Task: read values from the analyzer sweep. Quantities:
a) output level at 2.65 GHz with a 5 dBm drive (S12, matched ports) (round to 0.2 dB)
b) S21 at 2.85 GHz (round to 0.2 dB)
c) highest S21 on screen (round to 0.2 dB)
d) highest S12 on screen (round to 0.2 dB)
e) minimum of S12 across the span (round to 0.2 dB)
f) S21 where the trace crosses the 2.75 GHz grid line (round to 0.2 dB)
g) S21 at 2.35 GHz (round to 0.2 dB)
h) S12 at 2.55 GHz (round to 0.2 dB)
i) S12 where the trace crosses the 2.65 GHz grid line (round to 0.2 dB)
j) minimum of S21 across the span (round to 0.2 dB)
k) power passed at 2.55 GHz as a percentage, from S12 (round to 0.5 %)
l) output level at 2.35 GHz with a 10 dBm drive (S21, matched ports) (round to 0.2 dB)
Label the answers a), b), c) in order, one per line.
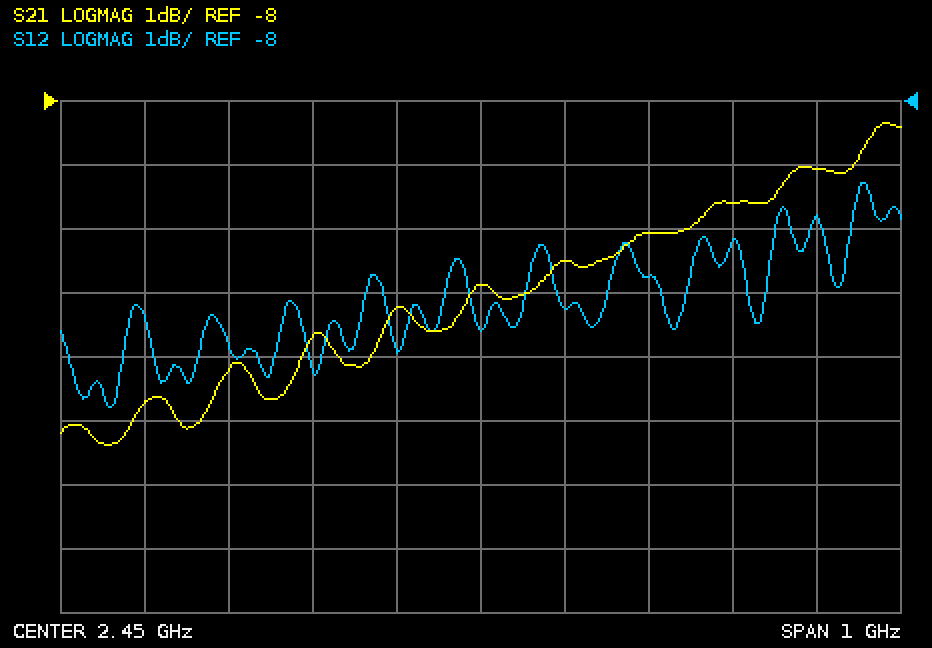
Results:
a) -5.8 dBm
b) -9.0 dB
c) -8.4 dB
d) -9.2 dB
e) -12.8 dB
f) -9.6 dB
g) -11.2 dB
h) -11.2 dB
i) -10.8 dB
j) -13.4 dB
k) 7.5 %
l) -1.2 dBm
